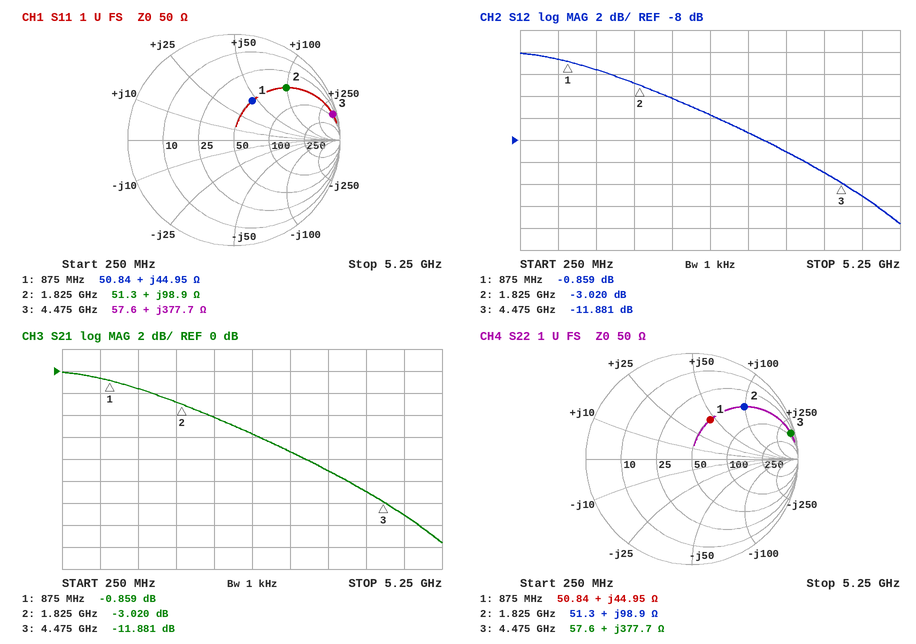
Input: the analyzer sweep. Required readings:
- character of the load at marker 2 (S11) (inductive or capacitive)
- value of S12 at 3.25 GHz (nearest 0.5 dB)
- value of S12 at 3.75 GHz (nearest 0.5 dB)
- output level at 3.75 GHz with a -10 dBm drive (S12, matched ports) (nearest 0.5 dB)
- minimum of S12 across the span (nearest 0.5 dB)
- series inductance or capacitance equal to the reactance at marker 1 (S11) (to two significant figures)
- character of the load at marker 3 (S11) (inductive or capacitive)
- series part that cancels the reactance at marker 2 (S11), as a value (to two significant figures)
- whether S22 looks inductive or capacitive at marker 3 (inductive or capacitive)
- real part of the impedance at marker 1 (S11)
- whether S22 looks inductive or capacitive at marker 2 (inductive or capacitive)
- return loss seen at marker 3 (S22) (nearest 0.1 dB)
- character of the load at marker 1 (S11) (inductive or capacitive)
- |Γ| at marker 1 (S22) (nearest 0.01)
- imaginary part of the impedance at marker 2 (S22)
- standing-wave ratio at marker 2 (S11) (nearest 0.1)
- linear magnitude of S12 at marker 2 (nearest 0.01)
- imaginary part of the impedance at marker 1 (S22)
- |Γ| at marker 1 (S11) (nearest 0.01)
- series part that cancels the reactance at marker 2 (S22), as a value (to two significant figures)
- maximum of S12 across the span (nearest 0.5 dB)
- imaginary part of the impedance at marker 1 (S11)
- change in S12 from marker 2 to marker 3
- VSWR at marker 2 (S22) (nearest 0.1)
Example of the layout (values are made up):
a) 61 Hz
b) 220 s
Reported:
a) inductive
b) -7.5 dB
c) -9.0 dB
d) -19.0 dBm
e) -15.5 dB
f) 8.2 nH
g) inductive
h) 880 fF
i) inductive
j) 50.84 Ω
k) inductive
l) 0.3 dB
m) inductive
n) 0.41
o) +98.9 Ω
p) 5.6
q) 0.71
r) +44.95 Ω
s) 0.41
t) 880 fF
u) 0.0 dB
v) +44.95 Ω
w) -8.861 dB
x) 5.6
